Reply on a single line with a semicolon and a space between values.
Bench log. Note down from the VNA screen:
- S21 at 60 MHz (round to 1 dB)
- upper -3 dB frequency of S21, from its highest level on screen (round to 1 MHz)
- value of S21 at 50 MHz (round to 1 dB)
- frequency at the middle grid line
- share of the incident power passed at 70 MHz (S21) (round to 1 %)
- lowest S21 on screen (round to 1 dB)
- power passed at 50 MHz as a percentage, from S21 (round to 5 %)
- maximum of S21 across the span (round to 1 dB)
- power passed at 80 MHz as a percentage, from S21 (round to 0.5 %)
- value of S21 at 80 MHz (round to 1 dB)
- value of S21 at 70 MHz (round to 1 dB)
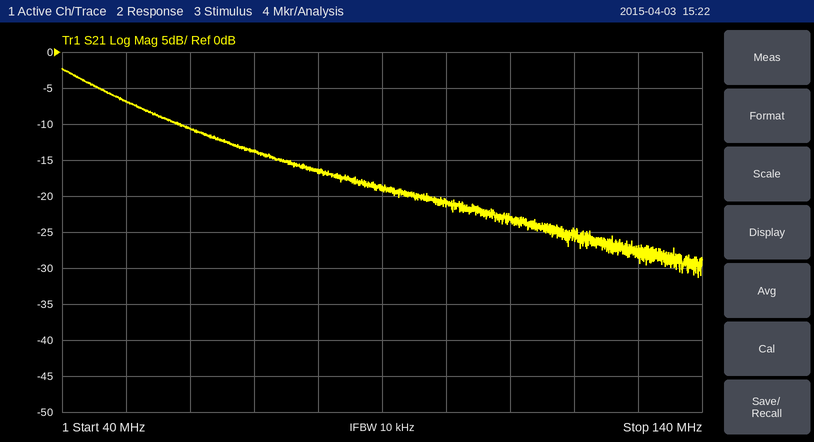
-11 dB; 46 MHz; -7 dB; 90 MHz; 4 %; -31 dB; 20 %; -2 dB; 2.0 %; -17 dB; -14 dB
